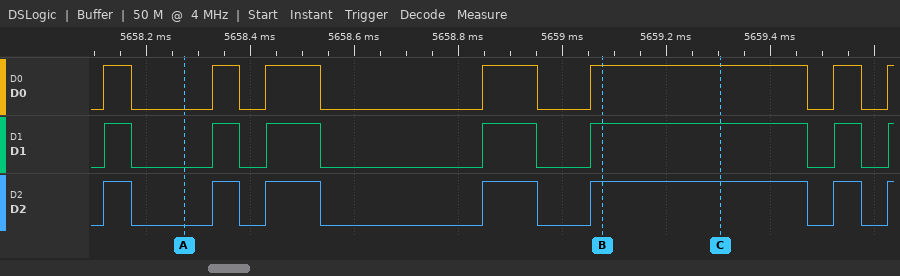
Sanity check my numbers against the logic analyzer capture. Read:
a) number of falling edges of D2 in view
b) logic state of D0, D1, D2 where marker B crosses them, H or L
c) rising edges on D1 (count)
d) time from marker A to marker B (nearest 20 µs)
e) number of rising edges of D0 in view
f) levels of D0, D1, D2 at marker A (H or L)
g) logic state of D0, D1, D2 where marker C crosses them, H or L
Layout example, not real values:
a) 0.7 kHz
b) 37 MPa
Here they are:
a) 6
b) D0=H, D1=H, D2=H
c) 7
d) 800 µs
e) 7
f) D0=L, D1=L, D2=L
g) D0=H, D1=H, D2=H
